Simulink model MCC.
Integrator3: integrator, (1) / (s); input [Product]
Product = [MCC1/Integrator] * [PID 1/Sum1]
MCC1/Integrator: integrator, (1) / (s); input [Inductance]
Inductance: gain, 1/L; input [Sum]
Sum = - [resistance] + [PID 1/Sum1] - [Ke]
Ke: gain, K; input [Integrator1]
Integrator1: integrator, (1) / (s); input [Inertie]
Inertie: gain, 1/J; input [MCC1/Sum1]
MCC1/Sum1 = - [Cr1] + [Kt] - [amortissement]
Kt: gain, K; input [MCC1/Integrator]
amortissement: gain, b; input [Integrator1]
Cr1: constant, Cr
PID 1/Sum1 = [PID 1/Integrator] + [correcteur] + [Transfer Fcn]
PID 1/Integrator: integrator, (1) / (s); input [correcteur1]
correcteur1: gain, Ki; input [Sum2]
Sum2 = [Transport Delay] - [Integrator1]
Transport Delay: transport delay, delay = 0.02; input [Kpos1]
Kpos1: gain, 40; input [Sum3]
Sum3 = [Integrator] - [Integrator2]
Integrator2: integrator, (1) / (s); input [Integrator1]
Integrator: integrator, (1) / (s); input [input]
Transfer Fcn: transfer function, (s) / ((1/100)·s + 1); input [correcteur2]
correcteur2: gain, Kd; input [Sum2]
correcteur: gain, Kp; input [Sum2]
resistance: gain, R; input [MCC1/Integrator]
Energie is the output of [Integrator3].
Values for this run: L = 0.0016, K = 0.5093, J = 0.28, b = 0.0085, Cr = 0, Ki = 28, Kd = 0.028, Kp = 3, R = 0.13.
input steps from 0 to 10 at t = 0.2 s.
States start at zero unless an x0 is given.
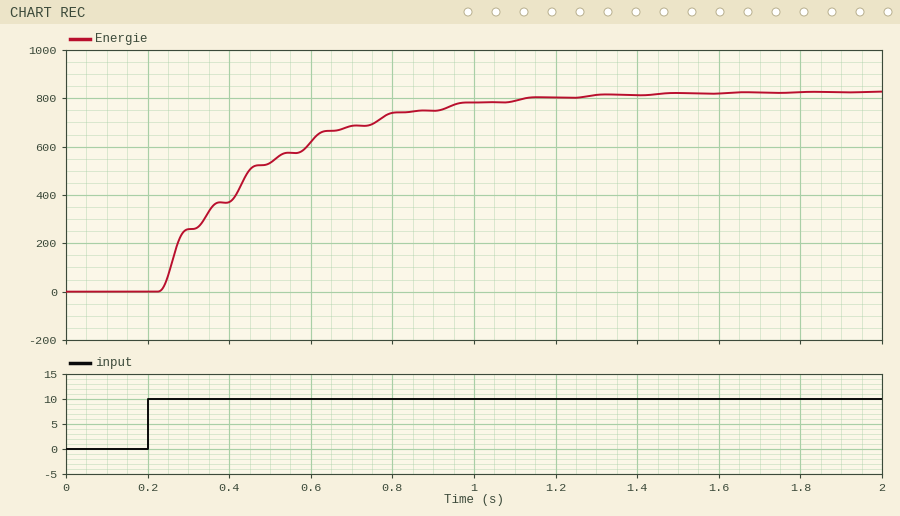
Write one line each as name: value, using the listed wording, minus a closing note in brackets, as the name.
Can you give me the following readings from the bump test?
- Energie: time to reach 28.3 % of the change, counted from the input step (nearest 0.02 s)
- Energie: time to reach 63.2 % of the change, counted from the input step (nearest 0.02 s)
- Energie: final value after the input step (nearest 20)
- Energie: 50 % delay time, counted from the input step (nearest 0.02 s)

Energie: time to reach 28.3 % of the change, counted from the input step: 0.08 s
Energie: time to reach 63.2 % of the change, counted from the input step: 0.26 s
Energie: final value after the input step: 820
Energie: 50 % delay time, counted from the input step: 0.22 s
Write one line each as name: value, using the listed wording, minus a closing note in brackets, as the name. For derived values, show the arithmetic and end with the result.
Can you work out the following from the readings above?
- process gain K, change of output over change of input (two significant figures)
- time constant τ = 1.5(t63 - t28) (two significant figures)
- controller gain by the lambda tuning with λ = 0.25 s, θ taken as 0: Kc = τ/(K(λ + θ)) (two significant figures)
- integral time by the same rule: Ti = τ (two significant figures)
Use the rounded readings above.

process gain K, change of output over change of input: (820 - 0) / 10 = 82
time constant τ = 1.5(t63 - t28): 1.5 × (0.26 - 0.08) = 0.27 s
controller gain by the lambda tuning with λ = 0.25 s, θ taken as 0: Kc = τ/(K(λ + θ)): 0.27 / (82 × (0.25 + 0)) = 0.013
integral time by the same rule: Ti = τ: 0.27 s
